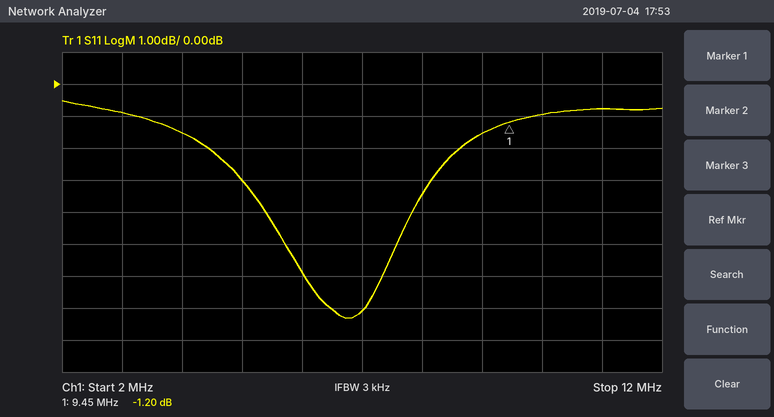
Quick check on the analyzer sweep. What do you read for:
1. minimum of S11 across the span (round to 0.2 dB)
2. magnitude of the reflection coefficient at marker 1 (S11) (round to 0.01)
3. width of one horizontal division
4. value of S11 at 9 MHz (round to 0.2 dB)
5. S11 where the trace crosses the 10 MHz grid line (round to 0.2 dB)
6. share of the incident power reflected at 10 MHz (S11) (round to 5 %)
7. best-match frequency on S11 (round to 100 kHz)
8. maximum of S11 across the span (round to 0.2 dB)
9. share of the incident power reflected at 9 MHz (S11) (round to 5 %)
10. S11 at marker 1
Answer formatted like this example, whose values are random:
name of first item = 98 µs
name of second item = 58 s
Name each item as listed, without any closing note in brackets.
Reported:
minimum of S11 across the span = -7.4 dB
magnitude of the reflection coefficient at marker 1 (S11) = 0.87
width of one horizontal division = 1 MHz
value of S11 at 9 MHz = -1.6 dB
S11 where the trace crosses the 10 MHz grid line = -1.0 dB
share of the incident power reflected at 10 MHz (S11) = 80 %
best-match frequency on S11 = 6.7 MHz
maximum of S11 across the span = -0.6 dB
share of the incident power reflected at 9 MHz (S11) = 70 %
S11 at marker 1 = -1.20 dB
